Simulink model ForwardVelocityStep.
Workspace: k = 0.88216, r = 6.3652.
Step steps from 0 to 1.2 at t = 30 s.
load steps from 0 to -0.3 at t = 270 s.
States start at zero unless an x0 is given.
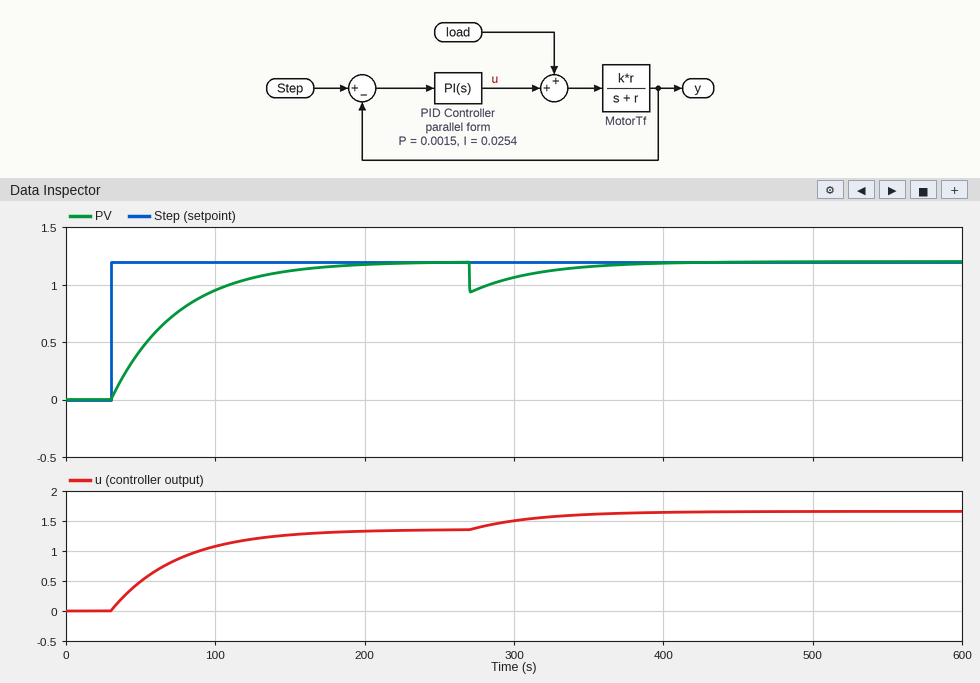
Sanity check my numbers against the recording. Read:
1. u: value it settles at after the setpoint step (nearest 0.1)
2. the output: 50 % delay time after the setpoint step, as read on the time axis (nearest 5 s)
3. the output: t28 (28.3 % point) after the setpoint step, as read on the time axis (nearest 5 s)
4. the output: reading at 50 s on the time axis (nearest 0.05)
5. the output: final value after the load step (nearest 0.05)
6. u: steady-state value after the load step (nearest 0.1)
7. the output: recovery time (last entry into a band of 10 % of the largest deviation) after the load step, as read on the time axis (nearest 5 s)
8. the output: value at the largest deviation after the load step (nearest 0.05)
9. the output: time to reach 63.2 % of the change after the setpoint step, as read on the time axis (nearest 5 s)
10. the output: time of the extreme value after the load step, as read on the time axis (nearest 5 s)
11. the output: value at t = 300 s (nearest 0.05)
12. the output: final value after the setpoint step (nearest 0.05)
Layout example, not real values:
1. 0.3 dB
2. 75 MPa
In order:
1. 1.4
2. 60 s
3. 45 s
4. 0.45
5. 1.20
6. 1.7
7. 375 s
8. 0.95
9. 75 s
10. 270 s
11. 1.05
12. 1.20
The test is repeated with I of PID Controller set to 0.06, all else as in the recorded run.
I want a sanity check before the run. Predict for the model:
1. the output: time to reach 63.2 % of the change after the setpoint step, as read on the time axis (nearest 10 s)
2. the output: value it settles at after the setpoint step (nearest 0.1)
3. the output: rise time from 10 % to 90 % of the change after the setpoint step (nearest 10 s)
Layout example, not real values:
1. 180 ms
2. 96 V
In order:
1. 50 s
2. 1.2
3. 40 s
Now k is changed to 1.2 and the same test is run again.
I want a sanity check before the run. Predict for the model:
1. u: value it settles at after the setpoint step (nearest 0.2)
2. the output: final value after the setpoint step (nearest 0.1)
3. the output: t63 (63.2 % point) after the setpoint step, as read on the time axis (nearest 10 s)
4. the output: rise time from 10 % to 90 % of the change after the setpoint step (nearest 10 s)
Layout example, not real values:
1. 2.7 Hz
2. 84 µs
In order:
1. 1.0
2. 1.2
3. 60 s
4. 70 s
